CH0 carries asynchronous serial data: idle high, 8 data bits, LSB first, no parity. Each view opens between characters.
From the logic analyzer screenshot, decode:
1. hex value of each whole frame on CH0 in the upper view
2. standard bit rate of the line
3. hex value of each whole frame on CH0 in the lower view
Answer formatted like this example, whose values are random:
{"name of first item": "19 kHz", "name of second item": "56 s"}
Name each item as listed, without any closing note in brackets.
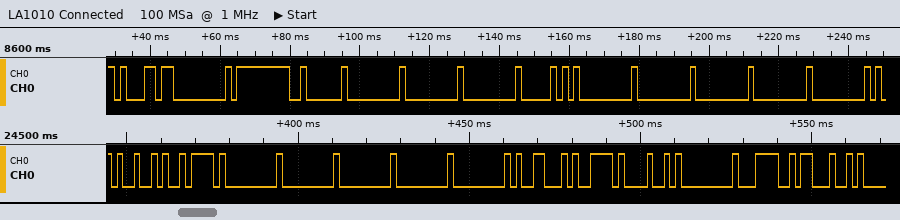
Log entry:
{"hex value of each whole frame on CH0 in the upper view": "B1, 00, FF, 02, 00, 00, 00, 50, 00, 00, 00, 00, 00", "standard bit rate of the line": "600 baud", "hex value of each whole frame on CH0 in the lower view": "49, 7A, 00, 00, 00, 00, 00, 19, 79, 48, 00, 3C, 23"}
